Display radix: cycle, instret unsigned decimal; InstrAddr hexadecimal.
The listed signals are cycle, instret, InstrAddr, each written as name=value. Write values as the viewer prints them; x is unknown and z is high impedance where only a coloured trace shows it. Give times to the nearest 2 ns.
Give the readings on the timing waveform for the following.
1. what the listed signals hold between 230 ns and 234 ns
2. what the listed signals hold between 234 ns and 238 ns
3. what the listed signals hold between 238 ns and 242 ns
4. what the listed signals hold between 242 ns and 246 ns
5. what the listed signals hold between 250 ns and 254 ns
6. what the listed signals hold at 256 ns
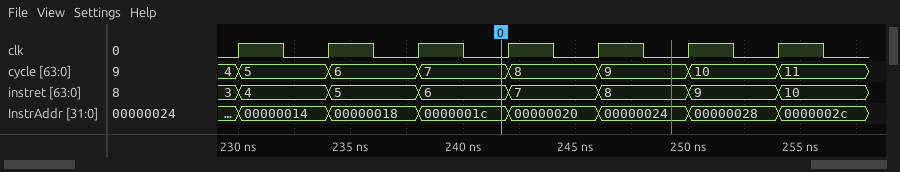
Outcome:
cycle=5, instret=4, InstrAddr=00000014
cycle=6, instret=5, InstrAddr=00000018
cycle=7, instret=6, InstrAddr=0000001c
cycle=8, instret=7, InstrAddr=00000020
cycle=10, instret=9, InstrAddr=00000028
cycle=11, instret=10, InstrAddr=0000002c
